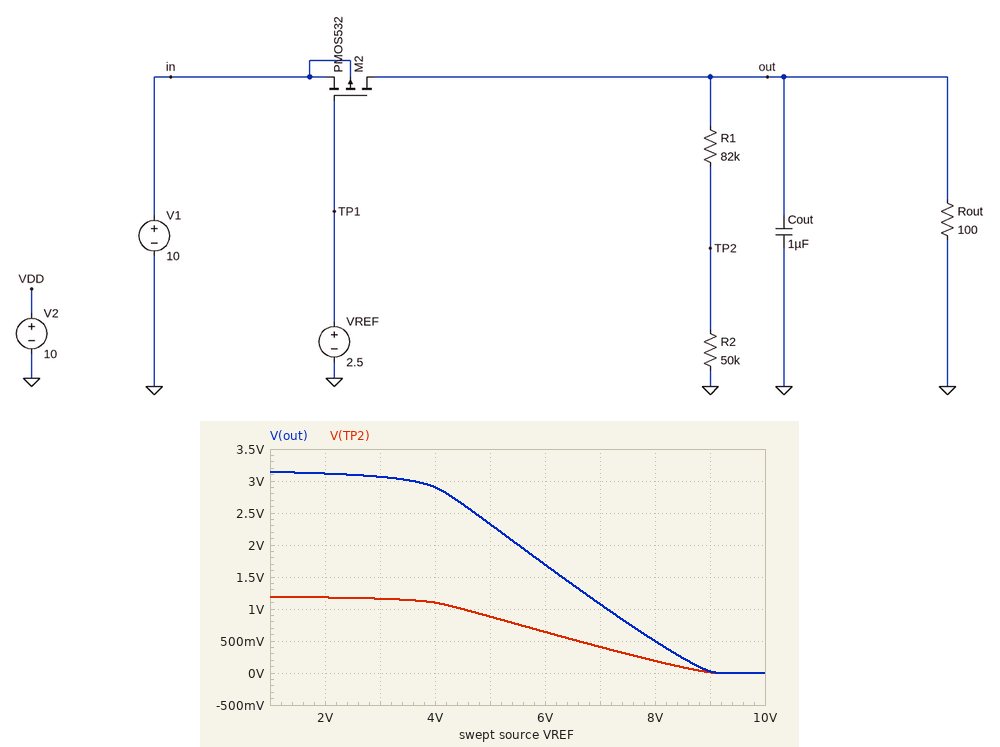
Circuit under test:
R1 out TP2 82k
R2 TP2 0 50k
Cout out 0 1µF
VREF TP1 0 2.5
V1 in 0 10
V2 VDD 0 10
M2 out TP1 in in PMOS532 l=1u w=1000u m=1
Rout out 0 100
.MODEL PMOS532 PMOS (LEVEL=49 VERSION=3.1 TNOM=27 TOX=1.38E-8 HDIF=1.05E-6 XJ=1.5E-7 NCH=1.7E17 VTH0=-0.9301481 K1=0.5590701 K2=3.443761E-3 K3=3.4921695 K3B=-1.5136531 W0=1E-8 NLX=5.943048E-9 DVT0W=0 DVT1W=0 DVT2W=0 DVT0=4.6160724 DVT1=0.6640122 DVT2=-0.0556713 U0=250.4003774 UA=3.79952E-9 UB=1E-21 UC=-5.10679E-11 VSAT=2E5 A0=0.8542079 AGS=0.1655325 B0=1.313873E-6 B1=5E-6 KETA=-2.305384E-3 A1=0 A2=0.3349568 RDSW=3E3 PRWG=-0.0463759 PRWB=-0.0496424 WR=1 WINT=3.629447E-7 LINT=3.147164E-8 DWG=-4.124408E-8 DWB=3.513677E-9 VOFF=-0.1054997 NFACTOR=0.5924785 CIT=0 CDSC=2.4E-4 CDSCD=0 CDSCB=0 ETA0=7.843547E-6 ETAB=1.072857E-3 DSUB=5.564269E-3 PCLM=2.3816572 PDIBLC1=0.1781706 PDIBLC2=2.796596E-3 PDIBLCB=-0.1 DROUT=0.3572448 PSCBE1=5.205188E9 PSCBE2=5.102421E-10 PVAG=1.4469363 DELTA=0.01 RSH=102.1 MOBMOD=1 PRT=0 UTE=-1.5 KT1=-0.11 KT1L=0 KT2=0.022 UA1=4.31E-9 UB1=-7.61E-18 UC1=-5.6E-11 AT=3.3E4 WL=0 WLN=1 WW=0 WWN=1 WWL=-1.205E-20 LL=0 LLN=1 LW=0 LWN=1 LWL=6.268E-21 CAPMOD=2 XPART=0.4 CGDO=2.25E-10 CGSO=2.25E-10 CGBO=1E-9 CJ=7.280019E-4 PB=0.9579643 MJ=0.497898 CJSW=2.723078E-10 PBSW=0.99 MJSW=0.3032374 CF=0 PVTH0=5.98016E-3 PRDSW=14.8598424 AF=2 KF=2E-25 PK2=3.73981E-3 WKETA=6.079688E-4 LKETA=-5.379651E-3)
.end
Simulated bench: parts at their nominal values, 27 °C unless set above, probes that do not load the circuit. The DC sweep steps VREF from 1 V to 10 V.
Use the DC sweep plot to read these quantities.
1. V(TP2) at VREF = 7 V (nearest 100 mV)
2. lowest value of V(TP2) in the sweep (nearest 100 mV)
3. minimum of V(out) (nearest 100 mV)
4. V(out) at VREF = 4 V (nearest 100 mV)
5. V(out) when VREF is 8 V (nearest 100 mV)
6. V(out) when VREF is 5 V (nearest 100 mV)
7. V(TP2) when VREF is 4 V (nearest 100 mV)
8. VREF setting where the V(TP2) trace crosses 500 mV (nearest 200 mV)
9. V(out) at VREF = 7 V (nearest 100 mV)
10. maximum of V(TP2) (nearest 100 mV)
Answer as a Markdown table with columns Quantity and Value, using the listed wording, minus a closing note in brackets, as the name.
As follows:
| Quantity | Value |
|---|---|
| V(TP2) at VREF = 7 V | 400 mV |
| lowest value of V(TP2) in the sweep | 0 V |
| minimum of V(out) | 0 V |
| V(out) at VREF = 4 V | 2.9 V |
| V(out) when VREF is 8 V | 500 mV |
| V(out) when VREF is 5 V | 2.3 V |
| V(TP2) when VREF is 4 V | 1.1 V |
| VREF setting where the V(TP2) trace crosses 500 mV | 6.6 V |
| V(out) at VREF = 7 V | 1.1 V |
| maximum of V(TP2) | 1.2 V |
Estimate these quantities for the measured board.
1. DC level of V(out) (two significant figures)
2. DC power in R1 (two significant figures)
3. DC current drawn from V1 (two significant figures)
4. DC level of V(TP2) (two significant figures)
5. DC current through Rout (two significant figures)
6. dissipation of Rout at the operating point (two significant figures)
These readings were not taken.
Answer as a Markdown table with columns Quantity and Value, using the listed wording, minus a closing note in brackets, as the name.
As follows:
| Quantity | Value |
|---|---|
| DC level of V(out) | 3.1 V |
| DC power in R1 | 45 µW |
| DC current drawn from V1 | 31 mA |
| DC level of V(TP2) | 1.2 V |
| DC current through Rout | 31 mA |
| dissipation of Rout at the operating point | 96 mW |
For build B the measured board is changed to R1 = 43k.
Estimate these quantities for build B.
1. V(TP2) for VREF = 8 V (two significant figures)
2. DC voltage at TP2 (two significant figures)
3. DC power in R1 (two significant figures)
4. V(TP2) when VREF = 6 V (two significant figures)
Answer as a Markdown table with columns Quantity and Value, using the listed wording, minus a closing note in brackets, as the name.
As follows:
| Quantity | Value |
|---|---|
| V(TP2) for VREF = 8 V | 270 mV |
| DC voltage at TP2 | 1.7 V |
| DC power in R1 | 48 µW |
| V(TP2) when VREF = 6 V | 910 mV |
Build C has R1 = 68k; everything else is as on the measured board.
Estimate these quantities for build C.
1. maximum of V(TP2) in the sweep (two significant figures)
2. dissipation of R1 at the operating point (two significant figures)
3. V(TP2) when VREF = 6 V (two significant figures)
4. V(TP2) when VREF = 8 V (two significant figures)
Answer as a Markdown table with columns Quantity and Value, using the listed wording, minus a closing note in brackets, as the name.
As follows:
| Quantity | Value |
|---|---|
| maximum of V(TP2) in the sweep | 1.3 V |
| dissipation of R1 at the operating point | 47 µW |
| V(TP2) when VREF = 6 V | 720 mV |
| V(TP2) when VREF = 8 V | 210 mV |
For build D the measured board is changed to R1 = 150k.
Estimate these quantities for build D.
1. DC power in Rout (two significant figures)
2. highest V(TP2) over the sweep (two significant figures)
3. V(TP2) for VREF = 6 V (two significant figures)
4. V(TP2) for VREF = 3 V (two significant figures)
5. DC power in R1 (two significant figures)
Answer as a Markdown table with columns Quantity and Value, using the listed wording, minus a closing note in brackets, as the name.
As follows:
| Quantity | Value |
|---|---|
| DC power in Rout | 96 mW |
| highest V(TP2) over the sweep | 790 mV |
| V(TP2) for VREF = 6 V | 420 mV |
| V(TP2) for VREF = 3 V | 770 mV |
| DC power in R1 | 36 µW |
